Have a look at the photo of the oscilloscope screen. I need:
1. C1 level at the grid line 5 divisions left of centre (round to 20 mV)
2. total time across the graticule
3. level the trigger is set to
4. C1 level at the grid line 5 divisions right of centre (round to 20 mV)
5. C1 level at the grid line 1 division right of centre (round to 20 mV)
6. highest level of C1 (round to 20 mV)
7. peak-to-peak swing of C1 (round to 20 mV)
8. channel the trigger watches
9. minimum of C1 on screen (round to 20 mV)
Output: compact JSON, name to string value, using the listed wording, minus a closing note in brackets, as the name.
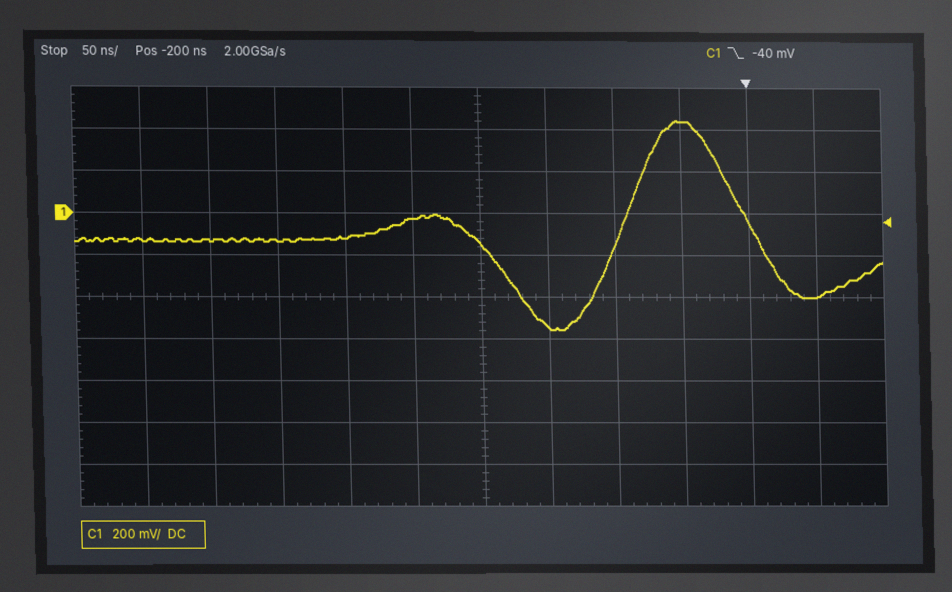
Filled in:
{"C1 level at the grid line 5 divisions left of centre": "-120 mV", "total time across the graticule": "600 ns", "level the trigger is set to": "-40 mV", "C1 level at the grid line 5 divisions right of centre": "-400 mV", "C1 level at the grid line 1 division right of centre": "-540 mV", "highest level of C1": "440 mV", "peak-to-peak swing of C1": "1.00 V", "channel the trigger watches": "C1", "minimum of C1 on screen": "-560 mV"}
